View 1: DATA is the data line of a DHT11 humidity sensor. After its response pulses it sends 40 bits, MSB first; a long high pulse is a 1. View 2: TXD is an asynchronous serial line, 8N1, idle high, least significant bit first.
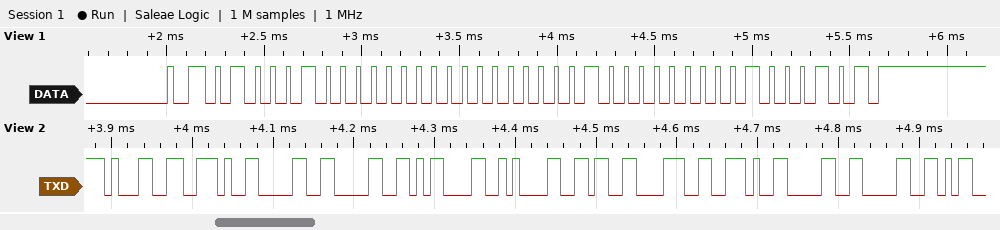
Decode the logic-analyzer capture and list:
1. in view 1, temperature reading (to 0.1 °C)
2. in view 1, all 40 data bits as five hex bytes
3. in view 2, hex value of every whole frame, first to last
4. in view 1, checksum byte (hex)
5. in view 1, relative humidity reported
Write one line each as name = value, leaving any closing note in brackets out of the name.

in view 1, temperature reading = 1.0 °C
in view 1, all 40 data bits as five hex bytes = 44 00 01 00 45
in view 2, hex value of every whole frame, first to last = 31 2E 30 30 0D 0A 36 38 2E 30 30
in view 1, checksum byte = 0x45
in view 1, relative humidity reported = 68 %
